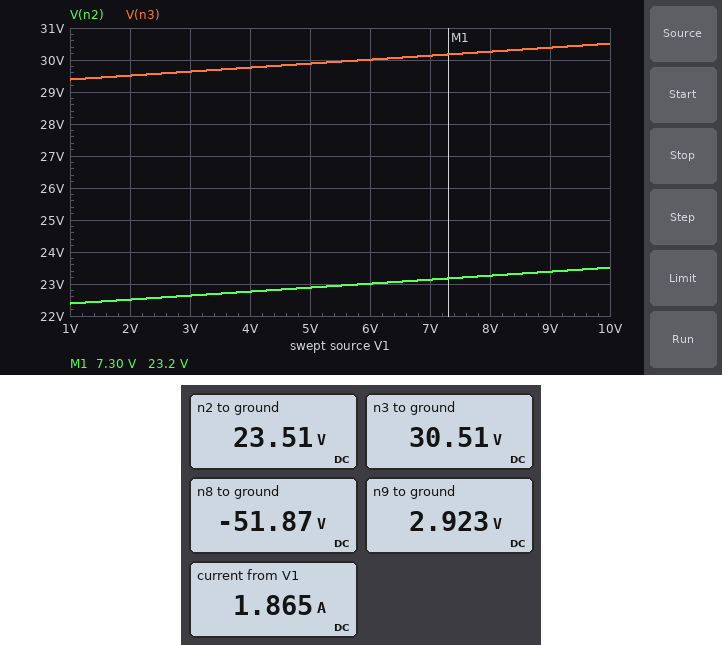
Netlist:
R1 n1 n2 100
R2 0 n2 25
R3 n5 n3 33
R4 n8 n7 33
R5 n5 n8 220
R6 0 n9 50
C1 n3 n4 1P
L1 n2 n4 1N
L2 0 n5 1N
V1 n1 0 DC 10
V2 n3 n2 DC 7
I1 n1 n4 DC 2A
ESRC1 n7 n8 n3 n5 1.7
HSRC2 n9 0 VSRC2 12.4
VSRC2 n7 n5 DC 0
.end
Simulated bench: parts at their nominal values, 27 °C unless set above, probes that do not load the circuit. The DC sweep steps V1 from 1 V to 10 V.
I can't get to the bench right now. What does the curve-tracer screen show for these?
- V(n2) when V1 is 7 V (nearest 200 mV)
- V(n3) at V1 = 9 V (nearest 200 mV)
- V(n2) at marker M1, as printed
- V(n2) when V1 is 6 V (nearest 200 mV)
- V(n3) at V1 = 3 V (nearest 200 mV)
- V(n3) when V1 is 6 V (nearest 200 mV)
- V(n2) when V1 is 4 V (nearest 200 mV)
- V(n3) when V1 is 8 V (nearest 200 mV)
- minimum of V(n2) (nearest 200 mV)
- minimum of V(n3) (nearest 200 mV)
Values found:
23.2 V
30.4 V
23.2 V
23.0 V
29.6 V
30.0 V
22.8 V
30.2 V
22.4 V
29.4 V
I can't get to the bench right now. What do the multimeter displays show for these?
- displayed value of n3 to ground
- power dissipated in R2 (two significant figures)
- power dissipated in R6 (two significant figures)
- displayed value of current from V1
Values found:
30.51 V
22 W
170 mW
1.865 A
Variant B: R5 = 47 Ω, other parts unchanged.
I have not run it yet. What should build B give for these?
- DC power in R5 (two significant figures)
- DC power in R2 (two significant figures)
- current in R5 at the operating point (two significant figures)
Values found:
57 W
22 W
1.1 A
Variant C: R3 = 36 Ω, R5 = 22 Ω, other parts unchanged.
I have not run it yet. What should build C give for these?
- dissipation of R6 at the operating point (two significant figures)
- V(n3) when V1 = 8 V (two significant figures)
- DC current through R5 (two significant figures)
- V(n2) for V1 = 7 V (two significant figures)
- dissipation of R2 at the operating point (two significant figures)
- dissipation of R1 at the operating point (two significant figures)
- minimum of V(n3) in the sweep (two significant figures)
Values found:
18 W
31 V
2.4 A
24 V
24 W
2.1 W
30 V
